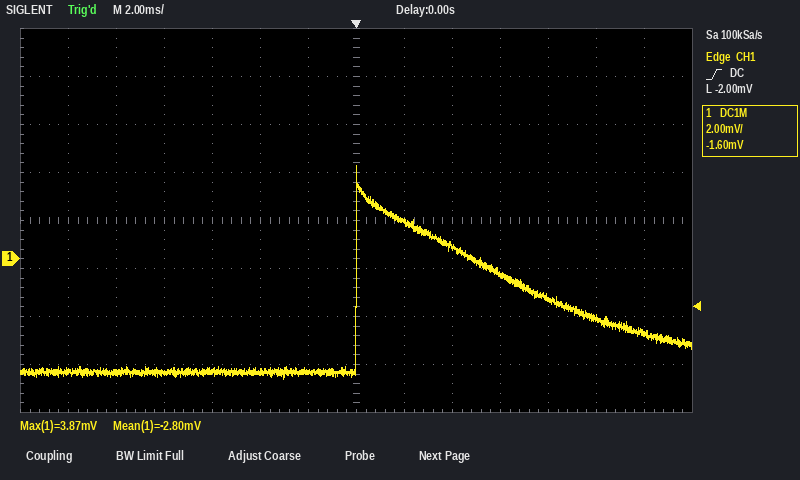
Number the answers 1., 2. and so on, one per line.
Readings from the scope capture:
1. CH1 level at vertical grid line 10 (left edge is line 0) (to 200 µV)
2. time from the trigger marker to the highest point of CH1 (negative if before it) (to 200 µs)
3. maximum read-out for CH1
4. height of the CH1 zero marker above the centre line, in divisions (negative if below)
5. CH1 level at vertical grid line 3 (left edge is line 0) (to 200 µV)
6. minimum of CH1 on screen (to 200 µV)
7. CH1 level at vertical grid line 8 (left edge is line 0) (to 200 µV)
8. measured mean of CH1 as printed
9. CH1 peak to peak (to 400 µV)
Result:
1. -600 µV
2. 0.0 ms
3. 3.87 mV
4. -0.8 div
5. -4.8 mV
6. -5.0 mV
7. 1.6 mV
8. -2.80 mV
9. 8.8 mV
